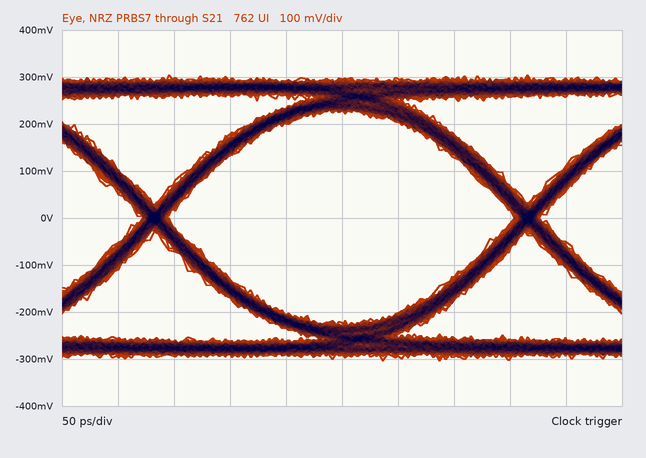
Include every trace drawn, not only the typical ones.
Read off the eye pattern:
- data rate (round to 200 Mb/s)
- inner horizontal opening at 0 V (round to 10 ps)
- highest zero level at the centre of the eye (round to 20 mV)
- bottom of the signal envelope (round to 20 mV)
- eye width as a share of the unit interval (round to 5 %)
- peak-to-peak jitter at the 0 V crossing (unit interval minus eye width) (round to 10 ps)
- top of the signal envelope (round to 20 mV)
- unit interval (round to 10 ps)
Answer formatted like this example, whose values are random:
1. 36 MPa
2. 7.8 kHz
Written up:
1. 3.0 Gb/s
2. 310 ps
3. -220 mV
4. -300 mV
5. 95 %
6. 20 ps
7. 300 mV
8. 330 ps
